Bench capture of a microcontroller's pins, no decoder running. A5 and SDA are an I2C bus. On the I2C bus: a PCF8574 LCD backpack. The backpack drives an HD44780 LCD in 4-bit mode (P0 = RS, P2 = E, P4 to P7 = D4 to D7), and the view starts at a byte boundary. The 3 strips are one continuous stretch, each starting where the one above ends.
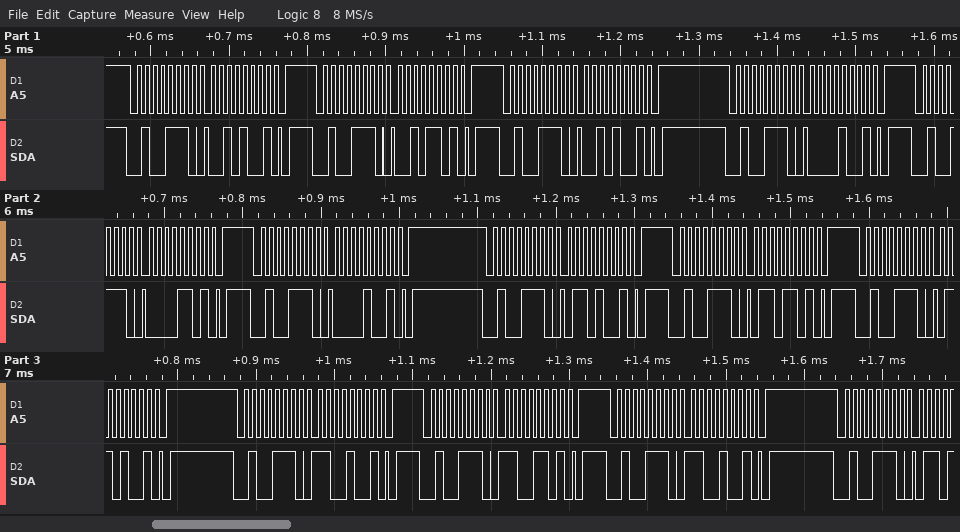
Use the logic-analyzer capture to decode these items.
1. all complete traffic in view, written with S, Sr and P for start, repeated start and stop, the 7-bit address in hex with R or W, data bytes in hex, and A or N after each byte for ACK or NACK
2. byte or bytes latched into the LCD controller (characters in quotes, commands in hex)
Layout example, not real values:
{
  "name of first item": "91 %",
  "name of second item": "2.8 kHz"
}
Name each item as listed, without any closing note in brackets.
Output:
{
  "all complete traffic in view, written with S, Sr and P for start, repeated start and stop, the 7-bit address in hex with R or W, data bytes in hex, and A or N after each byte for ACK or NACK": "S 27W A 29 A P S 27W A 2D A P S 27W A 29 A P S 27W A 09 A P S 27W A 0D A P S 27W A 09 A P S 27W A 69 A P S 27W A 6D A P S 27W A 69 A P S 27W A C9 A P S 27W A CD A P S 27W A C9 A P S 27W A",
  "byte or bytes latched into the LCD controller": "' ' 'l'"
}
